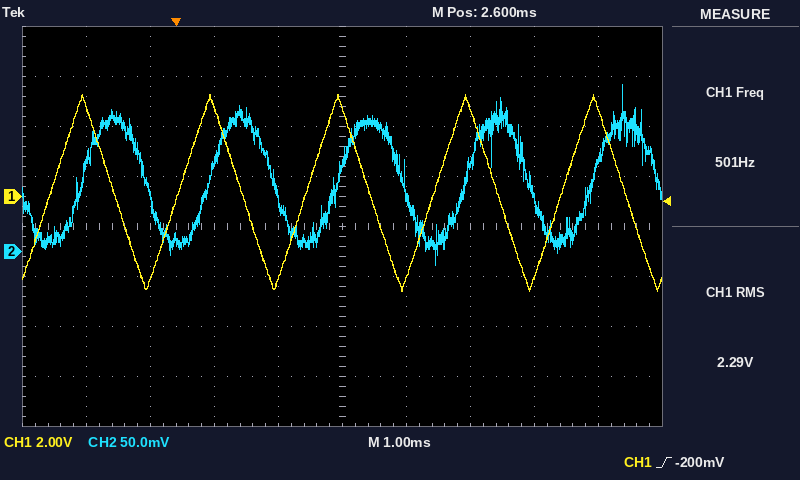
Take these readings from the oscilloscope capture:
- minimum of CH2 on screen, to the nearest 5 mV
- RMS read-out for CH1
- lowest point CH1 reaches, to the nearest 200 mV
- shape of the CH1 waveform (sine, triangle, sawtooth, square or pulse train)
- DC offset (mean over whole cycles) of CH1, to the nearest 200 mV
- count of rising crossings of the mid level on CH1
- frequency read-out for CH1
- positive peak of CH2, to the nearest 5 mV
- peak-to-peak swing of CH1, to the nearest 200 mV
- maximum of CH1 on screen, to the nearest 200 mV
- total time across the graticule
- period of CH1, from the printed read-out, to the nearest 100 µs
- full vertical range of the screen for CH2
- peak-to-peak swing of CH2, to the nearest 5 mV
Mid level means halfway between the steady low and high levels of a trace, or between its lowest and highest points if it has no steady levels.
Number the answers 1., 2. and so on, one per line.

1. -15 mV
2. 2.29 V
3. -3.8 V
4. triangle
5. 200 mV
6. 5
7. 501 Hz
8. 165 mV
9. 7.8 V
10. 4.0 V
11. 10 ms
12. 2.0 ms
13. 400 mV
14. 180 mV
